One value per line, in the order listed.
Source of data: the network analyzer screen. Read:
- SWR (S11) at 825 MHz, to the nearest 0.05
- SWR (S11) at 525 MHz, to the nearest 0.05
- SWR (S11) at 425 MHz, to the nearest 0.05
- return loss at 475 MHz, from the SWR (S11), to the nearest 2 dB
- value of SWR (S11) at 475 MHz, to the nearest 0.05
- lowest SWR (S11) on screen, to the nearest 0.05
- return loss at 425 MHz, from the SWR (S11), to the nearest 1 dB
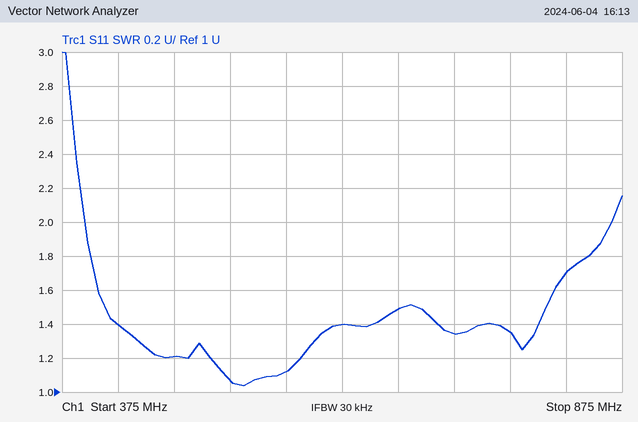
1.70
1.05
1.40
20 dB
1.20
1.05
16 dB
